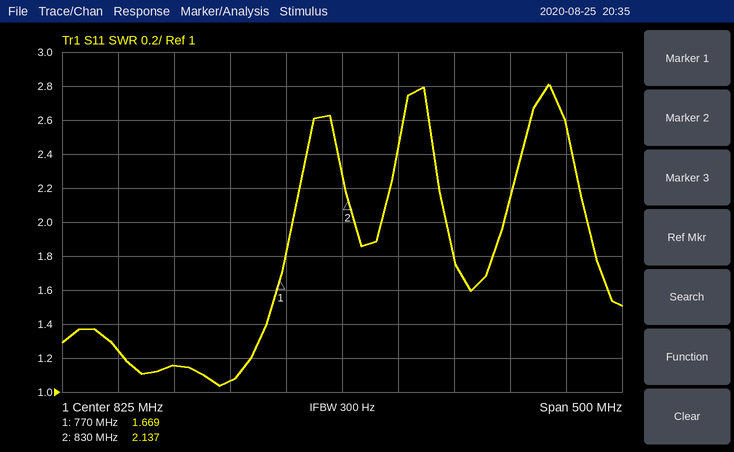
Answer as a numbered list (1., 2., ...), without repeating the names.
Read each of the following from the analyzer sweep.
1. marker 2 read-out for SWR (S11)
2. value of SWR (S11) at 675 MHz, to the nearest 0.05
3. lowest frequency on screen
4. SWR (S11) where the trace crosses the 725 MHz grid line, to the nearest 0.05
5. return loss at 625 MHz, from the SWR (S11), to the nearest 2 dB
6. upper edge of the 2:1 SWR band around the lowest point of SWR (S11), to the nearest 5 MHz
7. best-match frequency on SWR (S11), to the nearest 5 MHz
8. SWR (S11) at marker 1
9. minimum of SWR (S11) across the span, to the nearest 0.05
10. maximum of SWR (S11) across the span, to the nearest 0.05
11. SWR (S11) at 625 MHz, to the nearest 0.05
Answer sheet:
1. 2.137
2. 1.15
3. 575 MHz
4. 1.05
5. 20 dB
6. 780 MHz
7. 715 MHz
8. 1.669
9. 1.05
10. 2.80
11. 1.25
